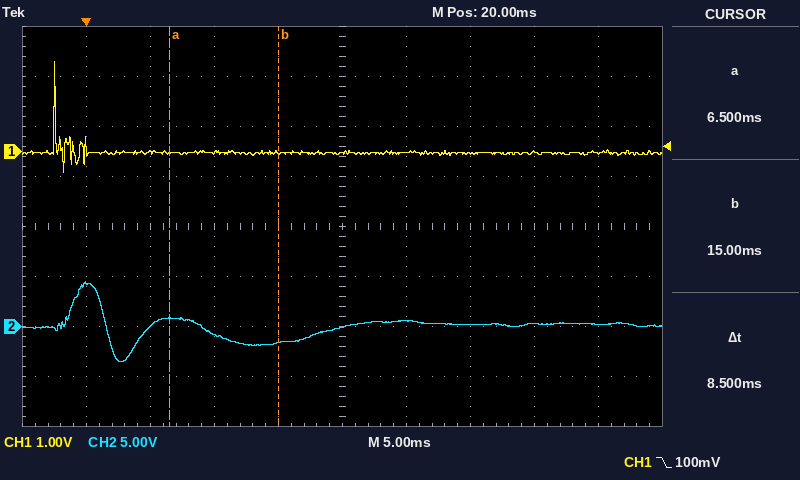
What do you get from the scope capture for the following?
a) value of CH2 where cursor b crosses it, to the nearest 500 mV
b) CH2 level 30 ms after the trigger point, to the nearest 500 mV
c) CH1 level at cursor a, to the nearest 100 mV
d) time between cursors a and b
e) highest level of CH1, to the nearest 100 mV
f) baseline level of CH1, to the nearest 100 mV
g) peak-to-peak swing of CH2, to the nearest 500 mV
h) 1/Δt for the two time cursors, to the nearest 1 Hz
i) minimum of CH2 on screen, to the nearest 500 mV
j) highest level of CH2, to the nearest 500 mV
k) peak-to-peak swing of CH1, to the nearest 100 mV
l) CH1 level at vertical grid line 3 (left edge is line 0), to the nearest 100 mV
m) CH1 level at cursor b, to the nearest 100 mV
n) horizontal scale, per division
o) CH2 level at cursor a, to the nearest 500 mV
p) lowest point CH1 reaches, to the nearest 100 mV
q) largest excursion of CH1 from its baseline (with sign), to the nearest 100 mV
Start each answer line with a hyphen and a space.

- -1.5 V
- 0.0 V
- 0.0 V
- 8.5 ms
- 1.8 V
- 0.0 V
- 8.0 V
- 118 Hz
- -3.5 V
- 4.5 V
- 2.2 V
- 0.0 V
- 0.0 V
- 5 ms
- 1.0 V
- -400 mV
- +1.8 V
